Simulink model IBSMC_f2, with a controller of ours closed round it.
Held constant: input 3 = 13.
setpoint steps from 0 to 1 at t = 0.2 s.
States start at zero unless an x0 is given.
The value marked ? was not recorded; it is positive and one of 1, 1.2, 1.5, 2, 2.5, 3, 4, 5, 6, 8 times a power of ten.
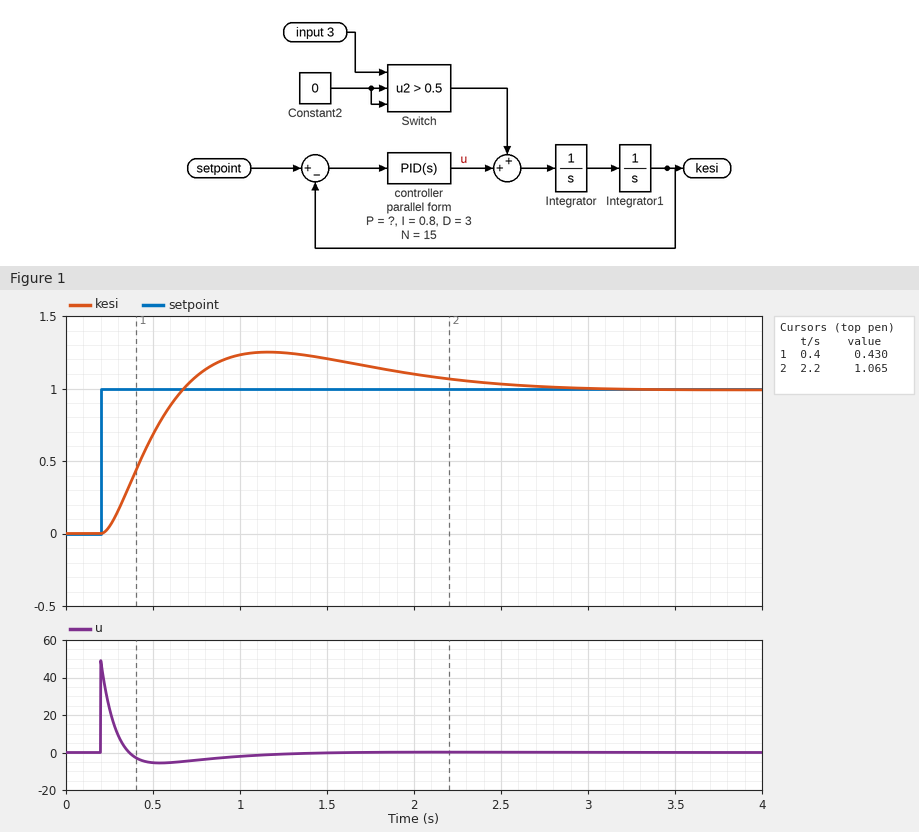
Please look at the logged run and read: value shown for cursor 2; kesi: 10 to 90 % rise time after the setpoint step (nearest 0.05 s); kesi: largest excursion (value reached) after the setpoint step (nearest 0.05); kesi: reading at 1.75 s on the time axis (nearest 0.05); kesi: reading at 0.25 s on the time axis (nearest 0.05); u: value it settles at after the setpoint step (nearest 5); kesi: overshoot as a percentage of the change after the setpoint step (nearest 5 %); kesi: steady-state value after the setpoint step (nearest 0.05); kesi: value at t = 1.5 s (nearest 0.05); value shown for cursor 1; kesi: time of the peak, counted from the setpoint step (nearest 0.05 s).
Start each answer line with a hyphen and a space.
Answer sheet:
- 1.065
- 0.35 s
- 1.25
- 1.15
- 0.05
- 0
- 25 %
- 1.00
- 1.20
- 0.430
- 0.95 s
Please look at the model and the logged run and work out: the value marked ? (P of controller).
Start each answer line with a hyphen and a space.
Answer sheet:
- 4
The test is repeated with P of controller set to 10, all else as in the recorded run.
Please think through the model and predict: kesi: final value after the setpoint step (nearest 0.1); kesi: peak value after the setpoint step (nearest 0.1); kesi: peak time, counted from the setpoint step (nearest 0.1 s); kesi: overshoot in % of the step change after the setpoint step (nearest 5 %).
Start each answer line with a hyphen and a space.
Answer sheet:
- 1.0
- 1.4
- 0.7 s
- 40 %
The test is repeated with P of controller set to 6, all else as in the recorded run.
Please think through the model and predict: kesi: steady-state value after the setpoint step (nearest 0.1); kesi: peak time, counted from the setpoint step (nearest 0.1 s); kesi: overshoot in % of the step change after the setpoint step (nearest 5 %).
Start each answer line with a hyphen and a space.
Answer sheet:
- 1.0
- 0.8 s
- 30 %
